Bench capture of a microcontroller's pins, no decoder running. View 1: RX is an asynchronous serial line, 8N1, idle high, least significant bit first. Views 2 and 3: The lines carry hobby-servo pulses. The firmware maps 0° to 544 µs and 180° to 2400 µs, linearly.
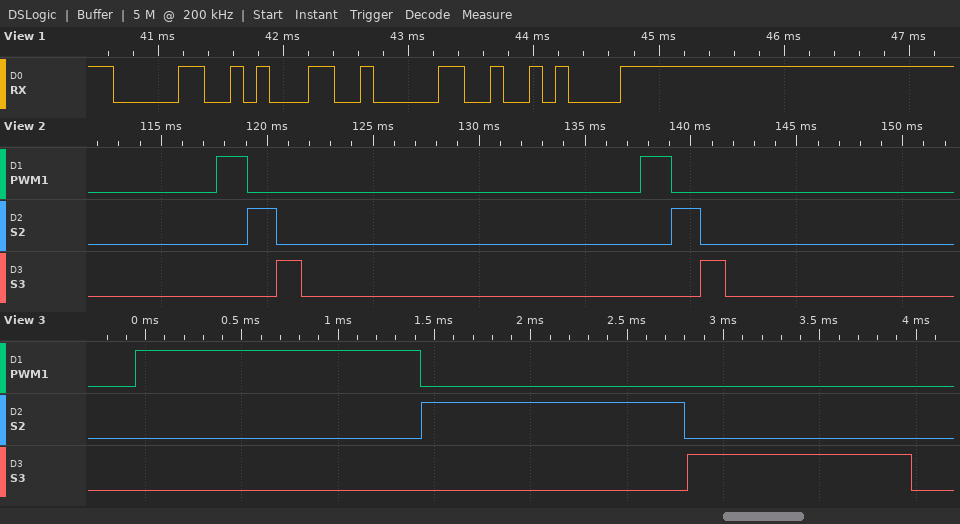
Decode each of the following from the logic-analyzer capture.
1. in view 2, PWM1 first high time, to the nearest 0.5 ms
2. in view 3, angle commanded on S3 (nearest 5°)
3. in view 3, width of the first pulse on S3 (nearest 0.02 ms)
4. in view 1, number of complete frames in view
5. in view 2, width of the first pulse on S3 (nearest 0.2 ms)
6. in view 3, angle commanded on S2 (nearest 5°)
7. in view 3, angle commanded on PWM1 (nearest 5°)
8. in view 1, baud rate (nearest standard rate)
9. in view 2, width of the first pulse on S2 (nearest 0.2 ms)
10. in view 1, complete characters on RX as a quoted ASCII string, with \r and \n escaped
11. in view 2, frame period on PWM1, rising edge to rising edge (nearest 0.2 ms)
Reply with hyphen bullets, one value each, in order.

- 1.5 ms
- 60°
- 1.16 ms
- 4
- 1.2 ms
- 80°
- 90°
- 9600 baud
- 1.4 ms
- "010\n"
- 20.0 ms
